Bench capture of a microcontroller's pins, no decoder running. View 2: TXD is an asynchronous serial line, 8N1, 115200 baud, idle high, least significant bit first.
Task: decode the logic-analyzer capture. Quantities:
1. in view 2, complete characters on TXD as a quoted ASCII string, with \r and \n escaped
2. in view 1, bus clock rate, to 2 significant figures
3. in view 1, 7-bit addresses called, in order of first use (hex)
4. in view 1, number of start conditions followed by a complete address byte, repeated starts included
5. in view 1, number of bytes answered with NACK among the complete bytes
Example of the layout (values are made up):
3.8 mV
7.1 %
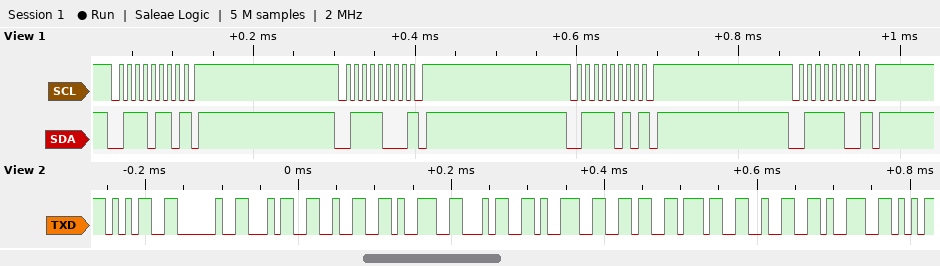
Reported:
"5 429496729"
100 kHz
0x3B 0x3C 0x3D 0x3E
4
4
